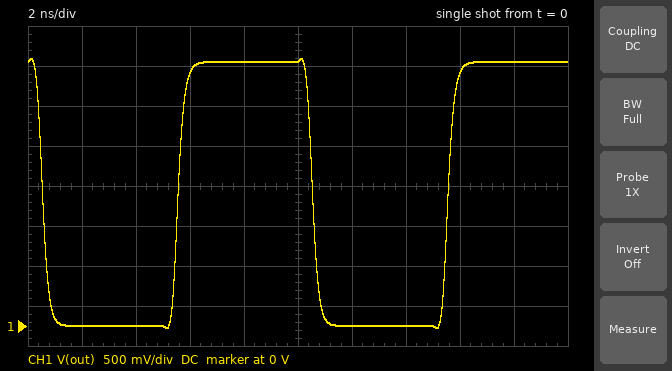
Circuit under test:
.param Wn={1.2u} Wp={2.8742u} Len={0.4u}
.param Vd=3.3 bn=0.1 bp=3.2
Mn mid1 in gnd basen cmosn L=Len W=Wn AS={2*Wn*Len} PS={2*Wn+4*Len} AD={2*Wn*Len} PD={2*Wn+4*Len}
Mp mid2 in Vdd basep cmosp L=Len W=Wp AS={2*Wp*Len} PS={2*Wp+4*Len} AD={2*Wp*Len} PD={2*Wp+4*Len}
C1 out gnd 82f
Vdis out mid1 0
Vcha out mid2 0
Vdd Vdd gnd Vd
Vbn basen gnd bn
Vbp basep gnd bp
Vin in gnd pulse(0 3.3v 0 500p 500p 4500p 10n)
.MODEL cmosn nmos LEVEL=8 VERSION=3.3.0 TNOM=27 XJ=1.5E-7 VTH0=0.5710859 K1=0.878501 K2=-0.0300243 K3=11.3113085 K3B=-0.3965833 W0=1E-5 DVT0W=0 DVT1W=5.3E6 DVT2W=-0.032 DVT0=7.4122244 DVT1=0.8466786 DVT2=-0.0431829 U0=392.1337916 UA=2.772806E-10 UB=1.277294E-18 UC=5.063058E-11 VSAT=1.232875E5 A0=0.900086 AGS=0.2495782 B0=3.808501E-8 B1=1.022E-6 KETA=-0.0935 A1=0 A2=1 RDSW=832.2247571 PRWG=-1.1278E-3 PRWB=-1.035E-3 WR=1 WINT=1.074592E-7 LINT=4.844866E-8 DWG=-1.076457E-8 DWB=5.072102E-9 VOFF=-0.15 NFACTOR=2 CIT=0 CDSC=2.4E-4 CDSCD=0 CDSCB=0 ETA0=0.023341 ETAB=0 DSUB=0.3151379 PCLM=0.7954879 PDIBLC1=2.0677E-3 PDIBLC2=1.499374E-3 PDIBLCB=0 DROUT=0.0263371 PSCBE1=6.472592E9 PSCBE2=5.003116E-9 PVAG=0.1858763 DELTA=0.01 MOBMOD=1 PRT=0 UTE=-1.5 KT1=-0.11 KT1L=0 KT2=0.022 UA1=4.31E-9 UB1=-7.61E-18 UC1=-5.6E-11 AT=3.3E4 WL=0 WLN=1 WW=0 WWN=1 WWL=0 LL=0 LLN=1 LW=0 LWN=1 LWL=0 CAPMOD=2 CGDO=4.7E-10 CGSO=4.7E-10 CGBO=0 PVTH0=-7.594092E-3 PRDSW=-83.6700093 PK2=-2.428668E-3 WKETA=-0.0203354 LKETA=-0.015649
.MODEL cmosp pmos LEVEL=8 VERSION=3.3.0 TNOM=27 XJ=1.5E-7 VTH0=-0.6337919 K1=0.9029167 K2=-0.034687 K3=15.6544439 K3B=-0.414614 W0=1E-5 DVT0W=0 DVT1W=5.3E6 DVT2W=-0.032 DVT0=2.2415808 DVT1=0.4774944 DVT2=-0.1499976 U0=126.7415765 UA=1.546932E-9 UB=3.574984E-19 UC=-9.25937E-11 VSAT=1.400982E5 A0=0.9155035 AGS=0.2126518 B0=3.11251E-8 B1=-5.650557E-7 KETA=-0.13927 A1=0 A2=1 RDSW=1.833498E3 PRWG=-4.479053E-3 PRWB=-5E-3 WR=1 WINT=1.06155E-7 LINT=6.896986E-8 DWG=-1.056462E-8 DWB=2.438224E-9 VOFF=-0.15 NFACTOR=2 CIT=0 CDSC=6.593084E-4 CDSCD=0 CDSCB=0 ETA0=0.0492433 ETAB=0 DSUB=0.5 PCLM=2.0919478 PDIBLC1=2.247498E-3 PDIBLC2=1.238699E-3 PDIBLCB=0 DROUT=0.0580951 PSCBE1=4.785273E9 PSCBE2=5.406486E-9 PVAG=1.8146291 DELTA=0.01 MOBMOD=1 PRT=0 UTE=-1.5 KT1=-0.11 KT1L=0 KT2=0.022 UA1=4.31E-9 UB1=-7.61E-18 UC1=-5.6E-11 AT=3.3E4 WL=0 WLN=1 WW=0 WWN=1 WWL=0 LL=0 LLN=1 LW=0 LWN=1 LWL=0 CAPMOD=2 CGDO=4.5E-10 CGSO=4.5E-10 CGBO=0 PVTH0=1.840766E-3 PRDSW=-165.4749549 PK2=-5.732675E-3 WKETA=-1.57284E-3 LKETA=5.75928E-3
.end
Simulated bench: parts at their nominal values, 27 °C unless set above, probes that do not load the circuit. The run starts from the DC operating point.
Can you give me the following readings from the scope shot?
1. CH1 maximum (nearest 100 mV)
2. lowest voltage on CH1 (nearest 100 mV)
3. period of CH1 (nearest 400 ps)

3.3 V
0 V
10.0 ns
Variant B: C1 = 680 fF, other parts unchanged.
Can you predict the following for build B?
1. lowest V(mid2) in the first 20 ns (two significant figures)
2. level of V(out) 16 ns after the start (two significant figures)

94 mV
810 mV
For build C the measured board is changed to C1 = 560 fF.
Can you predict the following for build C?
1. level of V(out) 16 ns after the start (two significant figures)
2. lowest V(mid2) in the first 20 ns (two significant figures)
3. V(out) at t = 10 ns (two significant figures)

910 mV
34 mV
3.2 V
